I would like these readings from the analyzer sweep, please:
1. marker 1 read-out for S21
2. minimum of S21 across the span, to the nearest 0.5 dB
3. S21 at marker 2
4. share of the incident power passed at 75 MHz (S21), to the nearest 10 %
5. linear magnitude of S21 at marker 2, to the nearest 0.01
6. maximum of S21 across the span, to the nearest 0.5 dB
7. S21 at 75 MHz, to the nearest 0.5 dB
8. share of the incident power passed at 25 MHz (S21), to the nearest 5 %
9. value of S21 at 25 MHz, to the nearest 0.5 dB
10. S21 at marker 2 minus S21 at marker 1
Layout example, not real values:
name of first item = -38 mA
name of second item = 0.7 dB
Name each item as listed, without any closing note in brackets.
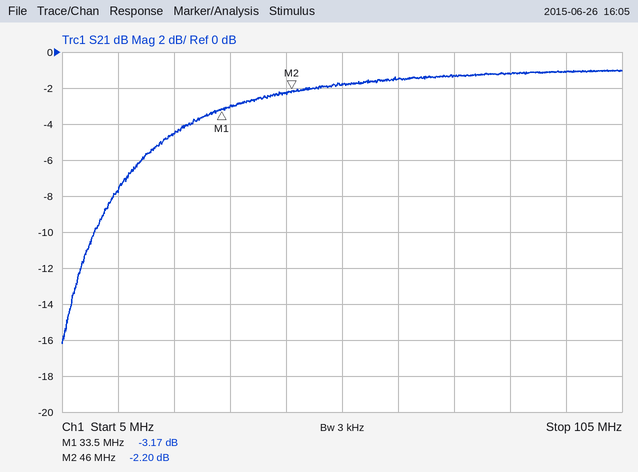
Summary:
marker 1 read-out for S21 = -3.17 dB
minimum of S21 across the span, to the nearest 0.5 dB = -16.0 dB
S21 at marker 2 = -2.20 dB
share of the incident power passed at 75 MHz (S21), to the nearest 10 % = 70 %
linear magnitude of S21 at marker 2, to the nearest 0.01 = 0.78
maximum of S21 across the span, to the nearest 0.5 dB = -1.0 dB
S21 at 75 MHz, to the nearest 0.5 dB = -1.5 dB
share of the incident power passed at 25 MHz (S21), to the nearest 5 % = 35 %
value of S21 at 25 MHz, to the nearest 0.5 dB = -4.5 dB
S21 at marker 2 minus S21 at marker 1 = 0.97 dB
